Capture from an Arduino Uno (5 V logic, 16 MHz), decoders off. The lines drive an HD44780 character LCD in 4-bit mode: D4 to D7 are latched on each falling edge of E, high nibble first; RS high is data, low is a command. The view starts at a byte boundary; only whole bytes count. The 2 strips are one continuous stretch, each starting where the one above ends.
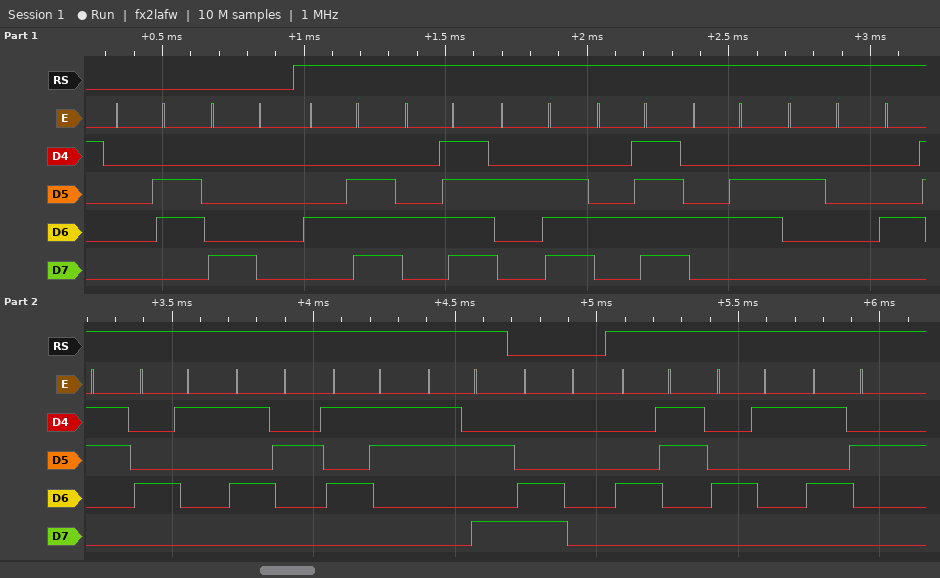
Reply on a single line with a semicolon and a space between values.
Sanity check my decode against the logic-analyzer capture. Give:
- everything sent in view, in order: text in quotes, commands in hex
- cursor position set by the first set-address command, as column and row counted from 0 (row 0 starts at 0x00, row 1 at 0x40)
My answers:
0x06 0x80 "NO.OF CARS:" 0xC0 "CAR"; column 0, row 0
